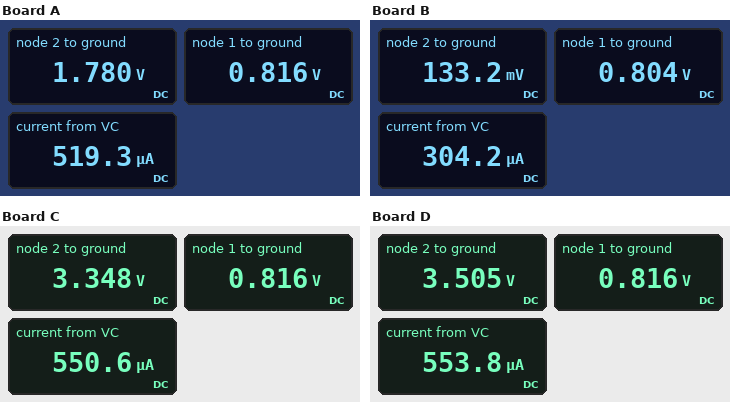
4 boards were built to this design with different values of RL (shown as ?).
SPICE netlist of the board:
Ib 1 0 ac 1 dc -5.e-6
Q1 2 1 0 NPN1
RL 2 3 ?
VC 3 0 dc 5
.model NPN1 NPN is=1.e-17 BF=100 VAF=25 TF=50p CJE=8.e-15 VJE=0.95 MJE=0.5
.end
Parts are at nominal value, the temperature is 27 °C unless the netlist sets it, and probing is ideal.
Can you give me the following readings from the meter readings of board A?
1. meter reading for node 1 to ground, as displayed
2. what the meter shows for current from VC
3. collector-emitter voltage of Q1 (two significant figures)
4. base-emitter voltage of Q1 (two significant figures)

0.816 V
519.3 µA
1.8 V
820 mV
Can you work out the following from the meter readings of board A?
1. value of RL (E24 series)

6.2 kΩ
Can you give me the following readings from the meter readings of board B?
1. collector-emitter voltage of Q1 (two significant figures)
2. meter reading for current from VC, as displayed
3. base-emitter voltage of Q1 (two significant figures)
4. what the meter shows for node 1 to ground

130 mV
304.2 µA
800 mV
0.804 V
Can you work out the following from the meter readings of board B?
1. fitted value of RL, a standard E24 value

16 kΩ
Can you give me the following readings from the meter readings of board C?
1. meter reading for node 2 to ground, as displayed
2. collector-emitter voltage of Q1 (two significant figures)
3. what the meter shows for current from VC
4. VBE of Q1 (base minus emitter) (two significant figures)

3.348 V
3.3 V
550.6 µA
820 mV
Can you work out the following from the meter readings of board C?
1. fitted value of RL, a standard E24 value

3 kΩ
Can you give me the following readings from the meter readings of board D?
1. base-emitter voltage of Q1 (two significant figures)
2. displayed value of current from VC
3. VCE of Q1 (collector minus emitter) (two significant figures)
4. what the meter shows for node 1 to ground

820 mV
553.8 µA
3.5 V
0.816 V
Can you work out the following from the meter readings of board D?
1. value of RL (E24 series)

2.7 kΩ
